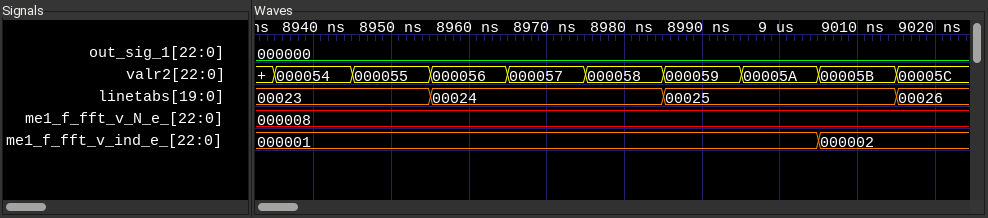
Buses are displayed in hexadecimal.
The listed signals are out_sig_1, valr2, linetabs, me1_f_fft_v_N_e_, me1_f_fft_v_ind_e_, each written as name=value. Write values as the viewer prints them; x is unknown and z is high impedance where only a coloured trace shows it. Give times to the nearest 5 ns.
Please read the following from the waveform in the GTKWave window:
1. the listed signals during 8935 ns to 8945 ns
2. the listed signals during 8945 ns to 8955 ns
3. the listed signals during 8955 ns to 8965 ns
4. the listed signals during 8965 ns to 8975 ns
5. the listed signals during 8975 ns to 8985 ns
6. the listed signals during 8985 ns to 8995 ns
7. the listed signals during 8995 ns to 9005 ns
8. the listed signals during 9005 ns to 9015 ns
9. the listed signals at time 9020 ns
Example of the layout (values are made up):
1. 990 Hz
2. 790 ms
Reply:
1. out_sig_1=000000, valr2=000054, linetabs=00023, me1_f_fft_v_N_e_=000008, me1_f_fft_v_ind_e_=000001
2. out_sig_1=000000, valr2=000055, linetabs=00023, me1_f_fft_v_N_e_=000008, me1_f_fft_v_ind_e_=000001
3. out_sig_1=000000, valr2=000056, linetabs=00024, me1_f_fft_v_N_e_=000008, me1_f_fft_v_ind_e_=000001
4. out_sig_1=000000, valr2=000057, linetabs=00024, me1_f_fft_v_N_e_=000008, me1_f_fft_v_ind_e_=000001
5. out_sig_1=000000, valr2=000058, linetabs=00024, me1_f_fft_v_N_e_=000008, me1_f_fft_v_ind_e_=000001
6. out_sig_1=000000, valr2=000059, linetabs=00025, me1_f_fft_v_N_e_=000008, me1_f_fft_v_ind_e_=000001
7. out_sig_1=000000, valr2=00005A, linetabs=00025, me1_f_fft_v_N_e_=000008, me1_f_fft_v_ind_e_=000001
8. out_sig_1=000000, valr2=00005B, linetabs=00025, me1_f_fft_v_N_e_=000008, me1_f_fft_v_ind_e_=000002
9. out_sig_1=000000, valr2=00005C, linetabs=00026, me1_f_fft_v_N_e_=000008, me1_f_fft_v_ind_e_=000002
